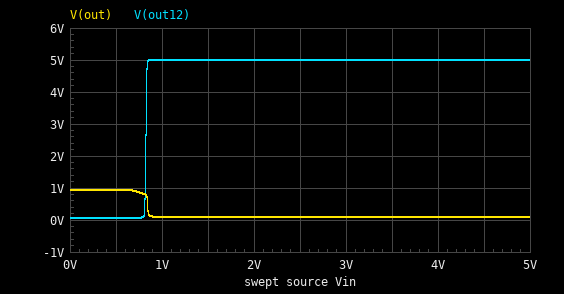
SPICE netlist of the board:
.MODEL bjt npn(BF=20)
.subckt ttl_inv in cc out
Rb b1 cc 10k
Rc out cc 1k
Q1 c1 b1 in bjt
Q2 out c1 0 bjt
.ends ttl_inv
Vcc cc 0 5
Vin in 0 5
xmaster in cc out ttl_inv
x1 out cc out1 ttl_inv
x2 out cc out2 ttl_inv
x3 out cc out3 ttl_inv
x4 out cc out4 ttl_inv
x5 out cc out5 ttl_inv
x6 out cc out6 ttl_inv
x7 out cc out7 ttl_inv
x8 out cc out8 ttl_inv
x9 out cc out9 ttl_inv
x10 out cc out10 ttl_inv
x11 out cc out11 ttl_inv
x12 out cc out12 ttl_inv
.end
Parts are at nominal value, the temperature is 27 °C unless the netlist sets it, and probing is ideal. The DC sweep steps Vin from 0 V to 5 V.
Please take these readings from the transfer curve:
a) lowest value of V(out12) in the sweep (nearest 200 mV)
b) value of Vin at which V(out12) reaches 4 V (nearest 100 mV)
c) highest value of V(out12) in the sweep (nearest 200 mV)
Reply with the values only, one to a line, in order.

0 V
800 mV
5.0 V
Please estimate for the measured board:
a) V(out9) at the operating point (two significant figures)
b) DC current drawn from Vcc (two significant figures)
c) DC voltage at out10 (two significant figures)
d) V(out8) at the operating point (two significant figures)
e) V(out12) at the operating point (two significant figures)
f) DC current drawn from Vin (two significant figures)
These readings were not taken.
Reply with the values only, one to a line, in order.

5.0 V
10 mA
5.0 V
5.0 V
5.0 V
340 µA
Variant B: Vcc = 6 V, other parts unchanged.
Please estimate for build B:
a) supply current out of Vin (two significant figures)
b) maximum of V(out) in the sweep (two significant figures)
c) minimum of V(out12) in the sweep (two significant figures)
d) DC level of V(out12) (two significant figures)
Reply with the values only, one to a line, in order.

440 µA
910 mV
67 mV
6.0 V
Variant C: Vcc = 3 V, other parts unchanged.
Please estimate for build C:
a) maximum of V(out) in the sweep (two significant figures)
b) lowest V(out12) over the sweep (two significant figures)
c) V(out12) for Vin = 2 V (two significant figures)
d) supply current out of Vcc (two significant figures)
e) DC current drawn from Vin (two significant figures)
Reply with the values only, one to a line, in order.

1.2 V
82 mV
3.0 V
5.5 mA
150 µA
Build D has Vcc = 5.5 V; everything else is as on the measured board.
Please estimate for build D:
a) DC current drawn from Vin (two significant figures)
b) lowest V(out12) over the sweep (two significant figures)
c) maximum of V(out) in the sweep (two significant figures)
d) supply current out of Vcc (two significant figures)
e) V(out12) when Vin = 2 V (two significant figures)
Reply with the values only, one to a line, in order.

390 µA
68 mV
920 mV
11 mA
5.5 V
